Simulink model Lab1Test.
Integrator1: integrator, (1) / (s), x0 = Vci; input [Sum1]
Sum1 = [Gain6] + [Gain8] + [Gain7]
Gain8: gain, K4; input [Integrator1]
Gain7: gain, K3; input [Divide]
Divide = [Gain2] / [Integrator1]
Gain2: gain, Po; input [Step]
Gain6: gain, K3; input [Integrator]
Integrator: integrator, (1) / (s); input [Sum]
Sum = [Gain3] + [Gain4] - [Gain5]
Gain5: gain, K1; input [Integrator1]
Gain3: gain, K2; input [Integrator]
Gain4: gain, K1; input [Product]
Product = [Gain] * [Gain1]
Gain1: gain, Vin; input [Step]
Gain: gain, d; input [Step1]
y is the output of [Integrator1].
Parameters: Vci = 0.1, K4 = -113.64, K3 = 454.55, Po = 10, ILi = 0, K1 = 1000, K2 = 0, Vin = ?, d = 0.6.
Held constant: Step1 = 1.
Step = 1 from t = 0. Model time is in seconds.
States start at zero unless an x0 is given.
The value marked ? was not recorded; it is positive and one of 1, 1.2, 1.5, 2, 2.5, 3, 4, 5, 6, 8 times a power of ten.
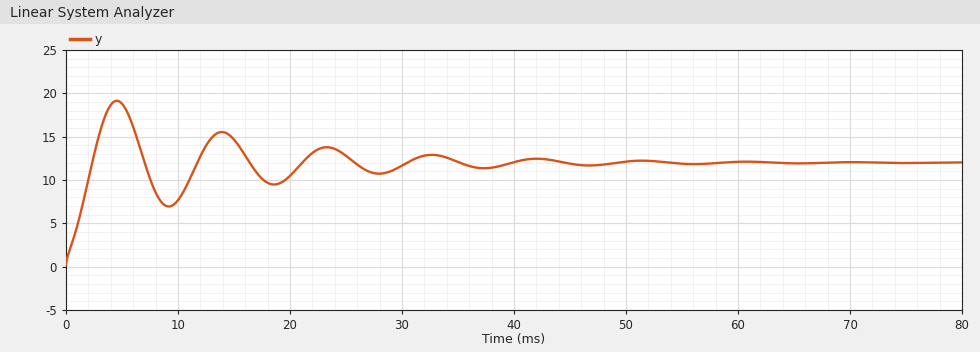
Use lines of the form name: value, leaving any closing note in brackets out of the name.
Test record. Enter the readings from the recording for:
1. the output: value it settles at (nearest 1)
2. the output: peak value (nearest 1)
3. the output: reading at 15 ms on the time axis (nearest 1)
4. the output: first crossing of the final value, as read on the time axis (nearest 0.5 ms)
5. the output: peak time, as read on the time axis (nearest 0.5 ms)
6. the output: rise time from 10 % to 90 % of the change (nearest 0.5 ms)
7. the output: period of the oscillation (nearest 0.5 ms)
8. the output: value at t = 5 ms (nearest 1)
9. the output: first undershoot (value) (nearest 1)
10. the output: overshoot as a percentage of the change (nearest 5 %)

the output: value it settles at: 12
the output: peak value: 19
the output: reading at 15 ms on the time axis: 15
the output: first crossing of the final value, as read on the time axis: 2.5 ms
the output: peak time, as read on the time axis: 4.5 ms
the output: rise time from 10 % to 90 % of the change: 2.0 ms
the output: period of the oscillation: 9.5 ms
the output: value at t = 5 ms: 19
the output: first undershoot (value): 7
the output: overshoot as a percentage of the change: 60 %
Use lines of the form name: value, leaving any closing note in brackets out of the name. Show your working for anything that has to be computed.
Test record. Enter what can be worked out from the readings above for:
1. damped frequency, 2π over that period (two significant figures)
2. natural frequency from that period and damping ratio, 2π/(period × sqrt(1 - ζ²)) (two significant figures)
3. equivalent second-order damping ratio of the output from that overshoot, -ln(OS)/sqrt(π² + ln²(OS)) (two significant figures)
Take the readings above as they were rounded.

damped frequency, 2π over that period: 2π / 9.5 = 0.66 rad/ms
natural frequency from that period and damping ratio, 2π/(period × sqrt(1 - ζ²)): 2π / (9.5 × sqrt(1 - 0.16²)) = 0.67 rad/ms
equivalent second-order damping ratio of the output from that overshoot, -ln(OS)/sqrt(π² + ln²(OS)): ln(0.6) = -0.511; 0.511 / sqrt(9.870 + 0.261) = 0.16
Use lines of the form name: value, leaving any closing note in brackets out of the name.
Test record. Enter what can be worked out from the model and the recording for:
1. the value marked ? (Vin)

the value marked ?: 20
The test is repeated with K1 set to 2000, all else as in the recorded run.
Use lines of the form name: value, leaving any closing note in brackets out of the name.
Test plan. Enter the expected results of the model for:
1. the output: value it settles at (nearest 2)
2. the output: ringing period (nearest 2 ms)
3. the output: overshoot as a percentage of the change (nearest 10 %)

the output: value it settles at: 12
the output: ringing period: 6 ms
the output: overshoot as a percentage of the change: 70 %
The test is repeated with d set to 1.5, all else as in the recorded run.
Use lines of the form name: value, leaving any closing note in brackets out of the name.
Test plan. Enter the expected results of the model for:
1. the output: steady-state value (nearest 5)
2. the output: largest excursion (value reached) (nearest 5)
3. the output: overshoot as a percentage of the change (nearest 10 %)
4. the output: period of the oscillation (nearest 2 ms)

the output: steady-state value: 30
the output: largest excursion (value reached): 50
the output: overshoot as a percentage of the change: 70 %
the output: period of the oscillation: 10 ms
